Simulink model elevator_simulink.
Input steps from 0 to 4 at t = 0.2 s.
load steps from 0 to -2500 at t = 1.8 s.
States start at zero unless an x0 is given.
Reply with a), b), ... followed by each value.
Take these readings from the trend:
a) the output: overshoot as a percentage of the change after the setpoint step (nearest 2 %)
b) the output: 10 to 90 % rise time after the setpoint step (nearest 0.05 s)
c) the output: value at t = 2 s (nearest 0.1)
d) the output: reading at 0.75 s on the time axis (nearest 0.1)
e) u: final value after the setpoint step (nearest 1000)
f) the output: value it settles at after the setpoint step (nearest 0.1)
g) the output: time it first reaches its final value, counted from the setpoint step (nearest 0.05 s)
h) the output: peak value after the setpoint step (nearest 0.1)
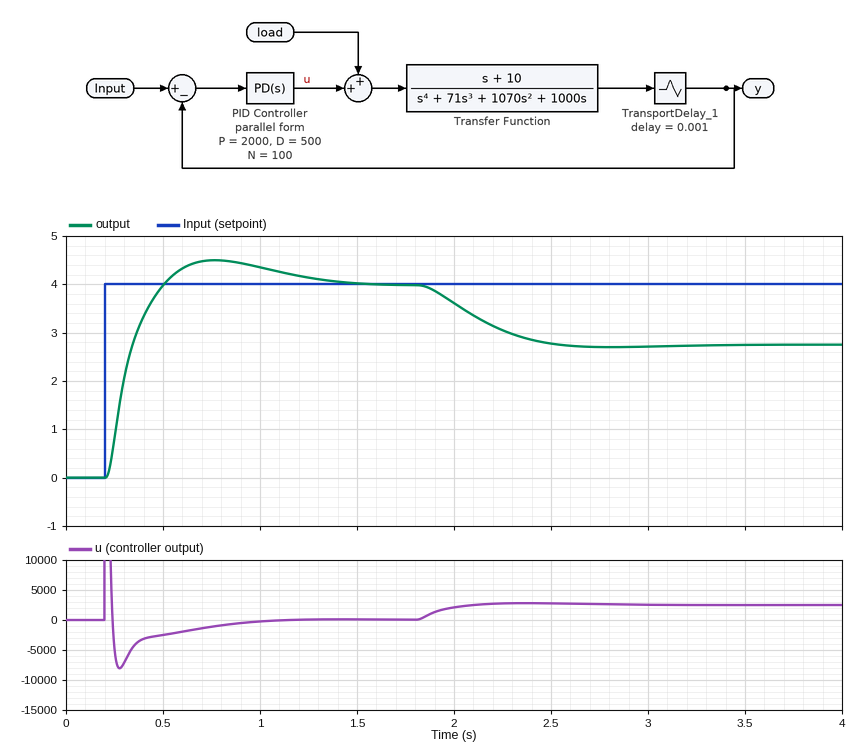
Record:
a) 12 %
b) 0.20 s
c) 3.6
d) 4.5
e) 0
f) 4.0
g) 0.30 s
h) 4.5
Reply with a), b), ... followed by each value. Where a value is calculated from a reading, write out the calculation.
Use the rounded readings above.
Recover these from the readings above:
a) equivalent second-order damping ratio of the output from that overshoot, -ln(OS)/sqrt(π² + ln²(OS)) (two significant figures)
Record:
a) ln(0.12) = -2.120; 2.120 / sqrt(9.870 + 4.496) = 0.56
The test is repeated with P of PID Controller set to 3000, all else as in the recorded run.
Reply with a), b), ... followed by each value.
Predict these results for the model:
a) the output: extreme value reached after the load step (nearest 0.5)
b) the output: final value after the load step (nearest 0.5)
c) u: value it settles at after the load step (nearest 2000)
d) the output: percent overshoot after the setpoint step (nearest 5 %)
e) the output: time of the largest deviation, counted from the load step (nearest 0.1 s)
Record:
a) 3.0
b) 3.0
c) 2000
d) 15 %
e) 0.7 s
